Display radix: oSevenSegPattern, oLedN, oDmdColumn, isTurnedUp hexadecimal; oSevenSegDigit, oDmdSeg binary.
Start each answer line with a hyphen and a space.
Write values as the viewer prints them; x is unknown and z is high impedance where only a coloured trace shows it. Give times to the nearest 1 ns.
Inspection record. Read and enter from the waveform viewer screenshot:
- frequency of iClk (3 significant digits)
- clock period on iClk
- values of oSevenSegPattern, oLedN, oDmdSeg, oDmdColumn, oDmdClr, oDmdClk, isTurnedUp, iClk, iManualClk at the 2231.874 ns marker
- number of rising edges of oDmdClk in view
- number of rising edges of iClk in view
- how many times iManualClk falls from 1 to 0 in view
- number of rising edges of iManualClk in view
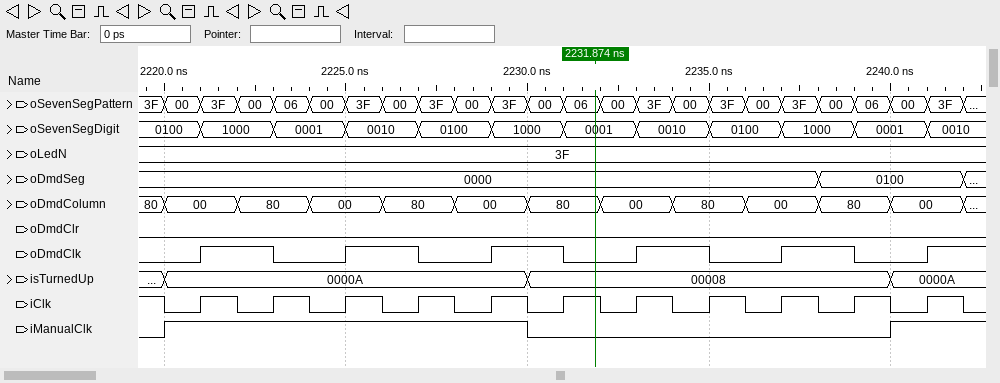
- 500 MHz
- 2 ns
- oSevenSegPattern=06, oLedN=3F, oDmdSeg=0000, oDmdColumn=80, oDmdClr=0, oDmdClk=0, isTurnedUp=00008, iClk=1, iManualClk=0
- 6
- 11
- 1
- 2
